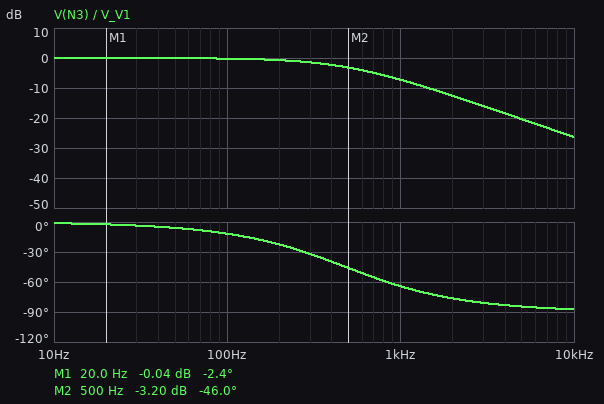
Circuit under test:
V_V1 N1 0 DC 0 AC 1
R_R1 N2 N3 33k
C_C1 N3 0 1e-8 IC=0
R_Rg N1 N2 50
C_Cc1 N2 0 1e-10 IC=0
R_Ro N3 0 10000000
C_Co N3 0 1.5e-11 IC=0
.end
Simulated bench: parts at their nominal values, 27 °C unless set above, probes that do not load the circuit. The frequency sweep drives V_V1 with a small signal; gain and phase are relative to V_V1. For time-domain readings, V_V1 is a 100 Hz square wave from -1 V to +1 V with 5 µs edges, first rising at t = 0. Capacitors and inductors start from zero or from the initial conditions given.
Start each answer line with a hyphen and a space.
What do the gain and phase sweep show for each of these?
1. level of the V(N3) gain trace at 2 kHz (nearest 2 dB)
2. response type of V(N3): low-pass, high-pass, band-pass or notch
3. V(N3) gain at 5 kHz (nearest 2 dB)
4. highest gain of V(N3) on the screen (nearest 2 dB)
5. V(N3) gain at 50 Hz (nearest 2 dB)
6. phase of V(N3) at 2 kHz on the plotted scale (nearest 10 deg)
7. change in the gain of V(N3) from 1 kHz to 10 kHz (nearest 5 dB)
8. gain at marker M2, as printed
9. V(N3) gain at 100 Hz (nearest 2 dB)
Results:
- -12 dB
- low-pass
- -20 dB
- 0 dB
- 0 dB
- -80 deg
- -20 dB
- -3.20 dB
- 0 dB
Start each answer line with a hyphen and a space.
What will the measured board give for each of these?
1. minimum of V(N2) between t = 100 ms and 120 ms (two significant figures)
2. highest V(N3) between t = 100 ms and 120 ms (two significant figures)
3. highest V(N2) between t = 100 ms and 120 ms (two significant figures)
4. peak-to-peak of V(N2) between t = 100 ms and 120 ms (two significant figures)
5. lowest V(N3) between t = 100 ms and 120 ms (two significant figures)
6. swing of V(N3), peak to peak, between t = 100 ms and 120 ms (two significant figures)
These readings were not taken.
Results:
- -1.0 V
- 1.0 V
- 1.0 V
- 2.0 V
- -1.0 V
- 2.0 V
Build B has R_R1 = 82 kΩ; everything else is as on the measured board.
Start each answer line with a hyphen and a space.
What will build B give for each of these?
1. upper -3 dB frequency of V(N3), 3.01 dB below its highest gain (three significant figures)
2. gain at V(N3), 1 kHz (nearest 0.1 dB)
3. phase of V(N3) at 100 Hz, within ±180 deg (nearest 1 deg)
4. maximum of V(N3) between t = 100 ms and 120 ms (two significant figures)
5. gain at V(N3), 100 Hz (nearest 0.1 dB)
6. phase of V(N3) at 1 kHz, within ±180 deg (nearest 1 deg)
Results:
- 195 Hz
- -14.4 dB
- -27 deg
- 990 mV
- -1.1 dB
- -79 deg
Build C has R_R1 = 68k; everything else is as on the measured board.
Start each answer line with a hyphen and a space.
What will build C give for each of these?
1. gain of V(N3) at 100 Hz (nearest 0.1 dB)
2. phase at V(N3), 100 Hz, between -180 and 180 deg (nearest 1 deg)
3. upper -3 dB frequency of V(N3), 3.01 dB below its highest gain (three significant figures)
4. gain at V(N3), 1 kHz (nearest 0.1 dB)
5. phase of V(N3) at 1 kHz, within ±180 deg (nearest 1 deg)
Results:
- -0.8 dB
- -23 deg
- 235 Hz
- -12.9 dB
- -77 deg
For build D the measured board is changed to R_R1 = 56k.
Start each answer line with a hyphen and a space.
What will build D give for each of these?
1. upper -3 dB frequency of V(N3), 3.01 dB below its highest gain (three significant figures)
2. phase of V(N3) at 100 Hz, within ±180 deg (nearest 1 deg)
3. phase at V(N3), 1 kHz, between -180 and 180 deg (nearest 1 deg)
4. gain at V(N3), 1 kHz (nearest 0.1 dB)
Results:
- 285 Hz
- -19 deg
- -74 deg
- -11.3 dB
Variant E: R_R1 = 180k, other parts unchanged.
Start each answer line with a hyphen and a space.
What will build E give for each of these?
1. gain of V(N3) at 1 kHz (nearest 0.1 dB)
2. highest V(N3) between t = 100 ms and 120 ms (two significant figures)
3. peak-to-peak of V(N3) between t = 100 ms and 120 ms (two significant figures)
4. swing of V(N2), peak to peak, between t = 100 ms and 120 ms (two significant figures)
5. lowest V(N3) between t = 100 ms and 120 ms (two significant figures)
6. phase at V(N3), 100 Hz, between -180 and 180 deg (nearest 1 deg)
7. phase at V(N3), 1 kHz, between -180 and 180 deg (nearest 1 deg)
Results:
- -21.1 dB
- 870 mV
- 1.7 V
- 2.0 V
- -870 mV
- -48 deg
- -85 deg
